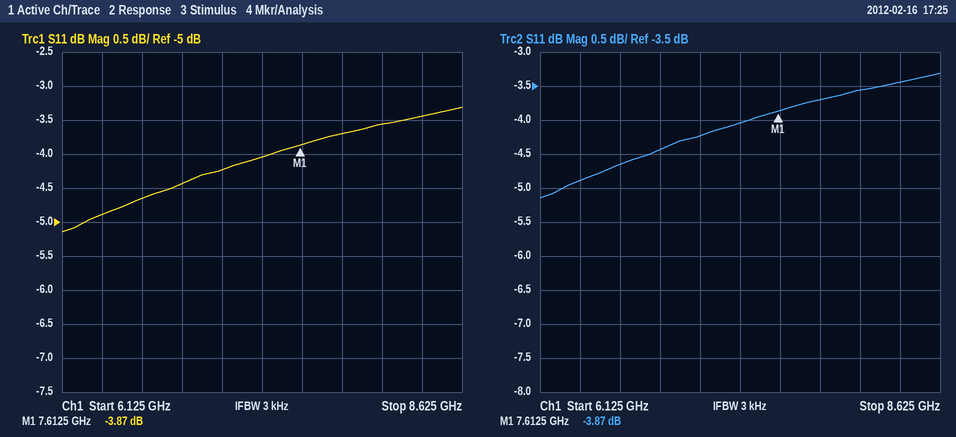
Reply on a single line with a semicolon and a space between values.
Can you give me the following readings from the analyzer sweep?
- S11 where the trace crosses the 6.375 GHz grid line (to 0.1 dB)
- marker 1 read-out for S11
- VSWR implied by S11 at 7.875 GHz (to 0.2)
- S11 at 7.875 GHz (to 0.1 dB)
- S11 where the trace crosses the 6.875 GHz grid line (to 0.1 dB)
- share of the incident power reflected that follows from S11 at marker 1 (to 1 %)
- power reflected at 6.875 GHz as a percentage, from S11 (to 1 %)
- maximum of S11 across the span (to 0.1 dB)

-4.9 dB; -3.87 dB; 4.8; -3.7 dB; -4.4 dB; 41 %; 36 %; -3.3 dB
